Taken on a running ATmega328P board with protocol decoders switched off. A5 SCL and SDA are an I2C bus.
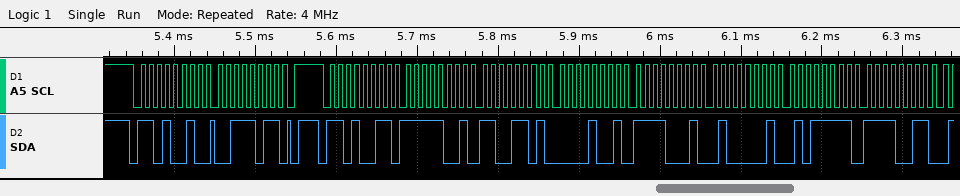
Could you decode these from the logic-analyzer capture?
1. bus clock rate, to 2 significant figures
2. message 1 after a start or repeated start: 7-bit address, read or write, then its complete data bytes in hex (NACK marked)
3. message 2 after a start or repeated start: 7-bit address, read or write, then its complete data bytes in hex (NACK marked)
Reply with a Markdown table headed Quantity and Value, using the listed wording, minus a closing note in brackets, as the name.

| Quantity | Value |
|---|---|
| bus clock rate, to 2 significant figures | 100 kHz |
| message 1 after a start or repeated start: 7-bit address, read or write, then its complete data bytes in hex | 0x69 write: 3B |
| message 2 after a start or repeated start: 7-bit address, read or write, then its complete data bytes in hex | 0x69 read: F9 CD 09 F1 41 5F F3 |
